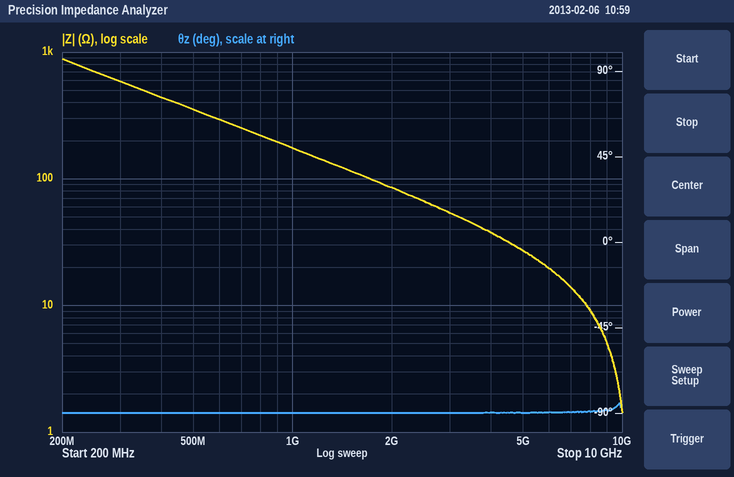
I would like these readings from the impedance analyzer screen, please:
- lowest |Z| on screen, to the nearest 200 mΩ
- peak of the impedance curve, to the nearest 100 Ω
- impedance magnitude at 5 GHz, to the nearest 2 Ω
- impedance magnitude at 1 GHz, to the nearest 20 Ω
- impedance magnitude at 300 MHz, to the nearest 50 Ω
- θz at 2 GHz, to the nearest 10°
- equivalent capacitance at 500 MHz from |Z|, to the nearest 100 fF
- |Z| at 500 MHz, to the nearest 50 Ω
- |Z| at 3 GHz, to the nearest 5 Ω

1.4 Ω
900 Ω
28 Ω
180 Ω
600 Ω
-90°
900 fF
350 Ω
55 Ω
